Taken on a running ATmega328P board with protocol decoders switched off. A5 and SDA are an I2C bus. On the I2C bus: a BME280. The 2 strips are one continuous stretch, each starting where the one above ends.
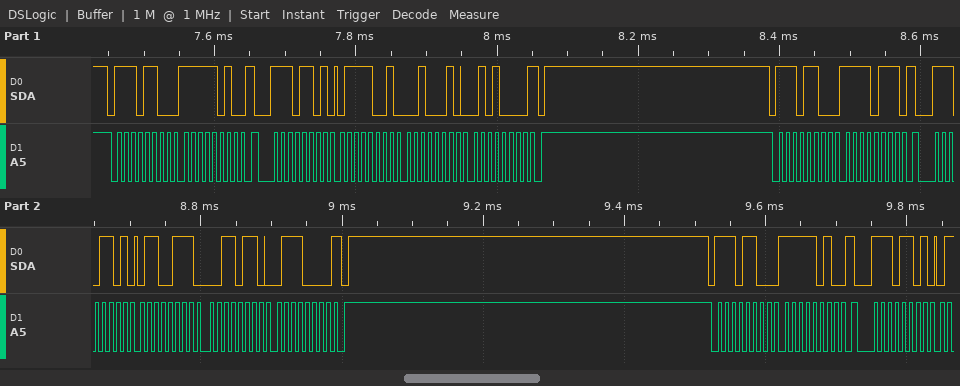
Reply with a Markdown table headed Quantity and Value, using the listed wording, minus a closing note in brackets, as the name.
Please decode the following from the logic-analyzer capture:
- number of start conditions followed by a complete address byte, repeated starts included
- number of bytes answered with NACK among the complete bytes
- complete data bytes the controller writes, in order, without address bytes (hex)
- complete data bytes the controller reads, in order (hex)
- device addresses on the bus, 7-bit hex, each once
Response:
| Quantity | Value |
|---|---|
| number of start conditions followed by a complete address byte, repeated starts included | 6 |
| number of bytes answered with NACK among the complete bytes | 2 |
| complete data bytes the controller writes, in order, without address bytes | FA F7 FA |
| complete data bytes the controller reads, in order | 79 22 50 67 36 70 |
| device addresses on the bus, 7-bit hex, each once | 0x76 |
